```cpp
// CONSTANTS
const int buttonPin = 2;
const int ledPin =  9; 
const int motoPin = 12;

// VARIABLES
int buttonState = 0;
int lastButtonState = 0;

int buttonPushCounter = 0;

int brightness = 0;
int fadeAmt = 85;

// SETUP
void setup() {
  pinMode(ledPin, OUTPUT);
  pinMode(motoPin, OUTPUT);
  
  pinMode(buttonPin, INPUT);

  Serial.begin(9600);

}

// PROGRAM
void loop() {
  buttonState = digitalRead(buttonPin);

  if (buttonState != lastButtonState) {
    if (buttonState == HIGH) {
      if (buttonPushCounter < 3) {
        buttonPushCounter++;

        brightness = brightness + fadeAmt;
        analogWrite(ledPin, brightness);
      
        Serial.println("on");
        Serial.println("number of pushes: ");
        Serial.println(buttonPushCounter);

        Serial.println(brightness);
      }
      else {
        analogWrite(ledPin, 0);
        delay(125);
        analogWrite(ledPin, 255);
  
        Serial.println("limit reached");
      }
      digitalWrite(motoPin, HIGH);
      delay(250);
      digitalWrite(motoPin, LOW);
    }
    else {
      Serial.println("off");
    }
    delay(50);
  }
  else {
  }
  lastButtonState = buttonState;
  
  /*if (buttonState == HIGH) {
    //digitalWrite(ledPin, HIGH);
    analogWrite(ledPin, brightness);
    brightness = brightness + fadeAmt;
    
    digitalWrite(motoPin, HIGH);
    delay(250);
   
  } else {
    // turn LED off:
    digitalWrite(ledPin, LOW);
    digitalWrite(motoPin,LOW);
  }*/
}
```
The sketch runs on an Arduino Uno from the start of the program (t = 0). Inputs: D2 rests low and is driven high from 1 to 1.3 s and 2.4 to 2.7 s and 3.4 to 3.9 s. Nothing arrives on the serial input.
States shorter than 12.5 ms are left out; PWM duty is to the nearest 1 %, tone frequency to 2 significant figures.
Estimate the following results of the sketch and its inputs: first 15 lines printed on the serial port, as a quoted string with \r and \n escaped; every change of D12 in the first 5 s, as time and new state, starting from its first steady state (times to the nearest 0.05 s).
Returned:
"on\r\nnumber of pushes: \r\n1\r\n85\r\noff\r\non\r\nnumber of pushes: \r\n2\r\n170\r\noff\r\non\r\nnumber of pushes: \r\n3\r\n255\r\noff\r\n"
0 s low; 1 s high; 1.25 s low; 2.4 s high; 2.65 s low; 3.4 s high; 3.65 s low
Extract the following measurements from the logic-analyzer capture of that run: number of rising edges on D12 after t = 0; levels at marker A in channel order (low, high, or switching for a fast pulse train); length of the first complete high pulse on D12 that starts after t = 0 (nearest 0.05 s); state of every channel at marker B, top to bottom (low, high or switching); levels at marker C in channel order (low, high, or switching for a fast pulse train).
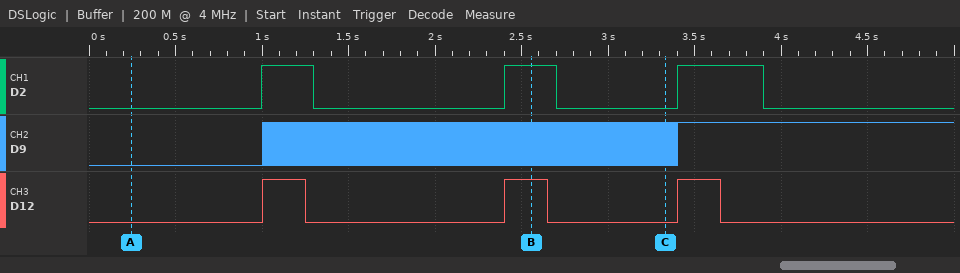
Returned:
3
D2 low, D9 low, D12 low
0.25 s
D2 high, D9 switching, D12 high
D2 low, D9 switching, D12 low
